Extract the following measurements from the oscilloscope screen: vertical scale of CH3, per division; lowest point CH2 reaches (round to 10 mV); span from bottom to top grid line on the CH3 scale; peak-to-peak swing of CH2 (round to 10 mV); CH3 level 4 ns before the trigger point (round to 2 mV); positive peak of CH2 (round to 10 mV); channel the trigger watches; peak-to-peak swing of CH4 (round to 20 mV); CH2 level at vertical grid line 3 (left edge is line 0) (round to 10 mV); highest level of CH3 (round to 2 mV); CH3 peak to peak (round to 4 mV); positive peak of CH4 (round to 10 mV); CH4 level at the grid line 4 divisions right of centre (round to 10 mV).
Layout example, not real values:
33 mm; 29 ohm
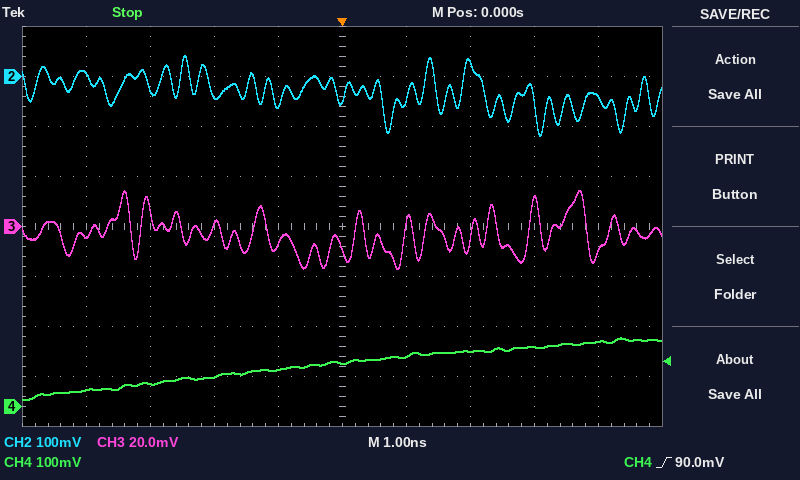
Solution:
20 mV; -120 mV; 160 mV; 160 mV; -4 mV; 40 mV; CH4; 120 mV; -40 mV; 14 mV; 32 mV; 140 mV; 130 mV
